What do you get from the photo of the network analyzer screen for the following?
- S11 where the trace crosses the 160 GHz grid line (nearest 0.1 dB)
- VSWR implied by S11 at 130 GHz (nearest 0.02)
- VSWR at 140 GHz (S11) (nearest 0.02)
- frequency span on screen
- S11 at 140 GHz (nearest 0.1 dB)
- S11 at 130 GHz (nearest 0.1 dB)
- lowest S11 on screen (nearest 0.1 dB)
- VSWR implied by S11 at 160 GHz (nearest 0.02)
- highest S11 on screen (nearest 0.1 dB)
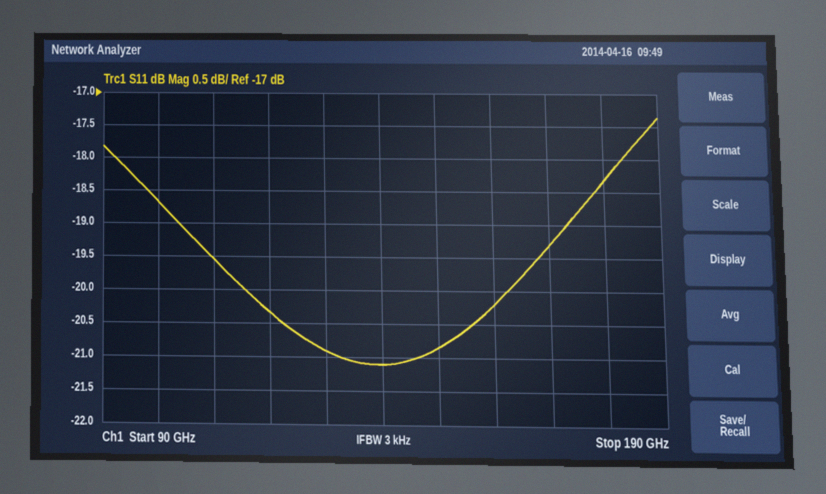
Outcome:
-20.2 dB
1.20
1.20
100 GHz
-21.1 dB
-20.9 dB
-21.1 dB
1.22
-17.4 dB
